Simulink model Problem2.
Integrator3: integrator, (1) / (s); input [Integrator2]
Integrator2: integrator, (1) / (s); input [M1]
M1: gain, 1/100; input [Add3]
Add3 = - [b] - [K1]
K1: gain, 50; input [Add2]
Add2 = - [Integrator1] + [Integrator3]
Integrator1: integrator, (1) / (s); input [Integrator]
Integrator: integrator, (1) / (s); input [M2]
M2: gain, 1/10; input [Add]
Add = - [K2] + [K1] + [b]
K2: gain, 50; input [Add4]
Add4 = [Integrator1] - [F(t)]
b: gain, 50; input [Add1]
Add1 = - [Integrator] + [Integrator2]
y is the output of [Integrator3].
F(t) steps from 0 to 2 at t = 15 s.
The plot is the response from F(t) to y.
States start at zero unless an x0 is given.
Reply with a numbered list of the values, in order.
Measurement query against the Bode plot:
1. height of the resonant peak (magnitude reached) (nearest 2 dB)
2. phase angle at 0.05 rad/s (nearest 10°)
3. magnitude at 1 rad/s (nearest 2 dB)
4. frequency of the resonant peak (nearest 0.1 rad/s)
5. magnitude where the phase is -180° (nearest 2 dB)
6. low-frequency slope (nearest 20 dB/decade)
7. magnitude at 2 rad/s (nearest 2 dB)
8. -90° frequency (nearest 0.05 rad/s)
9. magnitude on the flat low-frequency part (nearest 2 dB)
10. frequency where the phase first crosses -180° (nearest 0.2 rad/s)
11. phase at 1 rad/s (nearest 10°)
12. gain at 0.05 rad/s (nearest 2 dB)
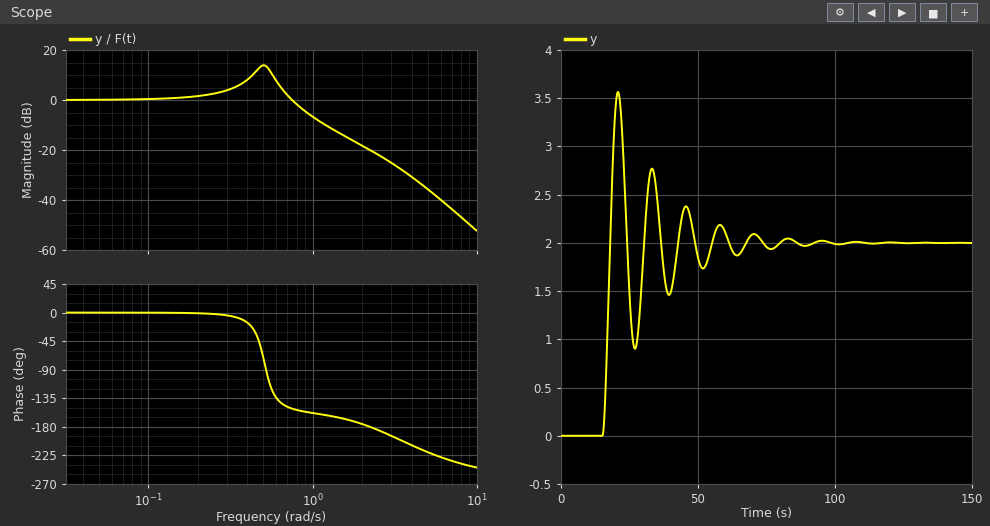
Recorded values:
1. 14 dB
2. 0°
3. -6 dB
4. 0.5 rad/s
5. -20 dB
6. 0 dB/decade
7. -18 dB
8. 0.50 rad/s
9. 0 dB
10. 2.2 rad/s
11. -160°
12. 0 dB
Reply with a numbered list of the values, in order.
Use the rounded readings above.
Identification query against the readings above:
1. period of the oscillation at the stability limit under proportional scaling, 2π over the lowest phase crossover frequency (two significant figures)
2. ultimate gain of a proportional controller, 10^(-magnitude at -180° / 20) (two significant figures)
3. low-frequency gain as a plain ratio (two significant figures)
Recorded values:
1. 2.9 s
2. 10
3. 1.0
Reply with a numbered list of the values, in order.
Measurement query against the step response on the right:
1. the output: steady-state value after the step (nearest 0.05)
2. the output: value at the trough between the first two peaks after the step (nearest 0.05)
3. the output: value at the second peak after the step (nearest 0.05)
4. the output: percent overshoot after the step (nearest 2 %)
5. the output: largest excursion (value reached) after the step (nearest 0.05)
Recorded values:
1. 2.00
2. 0.90
3. 2.75
4. 78 %
5. 3.55
